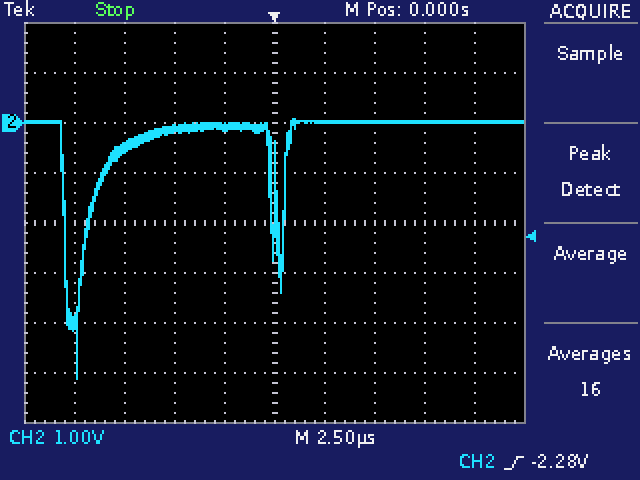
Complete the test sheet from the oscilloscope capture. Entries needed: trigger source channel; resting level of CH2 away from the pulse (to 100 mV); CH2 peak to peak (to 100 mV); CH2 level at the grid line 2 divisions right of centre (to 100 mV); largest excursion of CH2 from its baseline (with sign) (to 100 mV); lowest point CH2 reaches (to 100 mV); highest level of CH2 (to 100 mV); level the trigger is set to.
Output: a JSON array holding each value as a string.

["CH2", "0.0 V", "5.2 V", "0.0 V", "-5.1 V", "-5.1 V", "100 mV", "-2.28 V"]
